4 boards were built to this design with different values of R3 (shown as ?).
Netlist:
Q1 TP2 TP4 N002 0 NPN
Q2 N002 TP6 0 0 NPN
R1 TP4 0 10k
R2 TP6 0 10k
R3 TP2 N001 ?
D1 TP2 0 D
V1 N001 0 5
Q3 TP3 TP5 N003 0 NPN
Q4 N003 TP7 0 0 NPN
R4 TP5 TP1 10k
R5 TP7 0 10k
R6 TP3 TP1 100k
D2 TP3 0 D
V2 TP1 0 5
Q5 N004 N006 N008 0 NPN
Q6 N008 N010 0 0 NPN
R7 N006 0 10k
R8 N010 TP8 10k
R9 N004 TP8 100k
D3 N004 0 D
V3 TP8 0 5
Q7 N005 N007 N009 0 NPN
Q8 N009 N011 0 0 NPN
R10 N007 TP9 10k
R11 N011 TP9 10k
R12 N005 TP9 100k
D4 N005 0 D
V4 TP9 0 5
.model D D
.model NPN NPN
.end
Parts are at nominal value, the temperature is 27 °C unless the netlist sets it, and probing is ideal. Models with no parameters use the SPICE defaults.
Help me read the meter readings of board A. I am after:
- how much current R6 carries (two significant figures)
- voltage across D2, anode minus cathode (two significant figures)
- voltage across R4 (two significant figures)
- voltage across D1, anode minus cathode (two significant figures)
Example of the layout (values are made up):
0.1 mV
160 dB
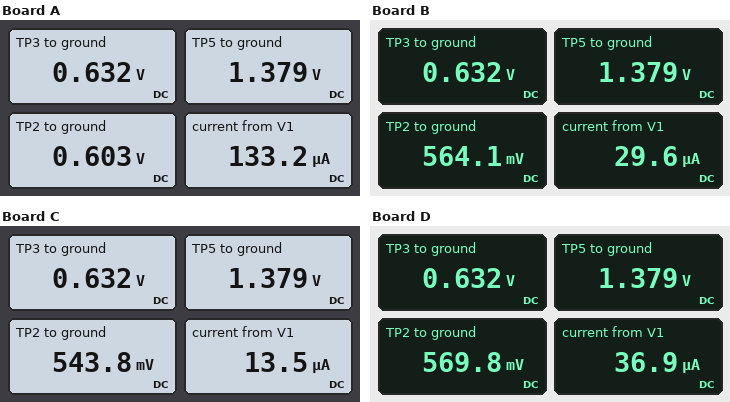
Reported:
44 µA
630 mV
3.6 V
600 mV
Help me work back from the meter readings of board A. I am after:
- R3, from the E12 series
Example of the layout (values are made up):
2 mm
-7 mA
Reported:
33 kΩ
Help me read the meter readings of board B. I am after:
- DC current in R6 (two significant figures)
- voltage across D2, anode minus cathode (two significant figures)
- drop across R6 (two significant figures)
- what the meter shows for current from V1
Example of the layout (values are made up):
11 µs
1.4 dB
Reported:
44 µA
630 mV
4.4 V
29.6 µA
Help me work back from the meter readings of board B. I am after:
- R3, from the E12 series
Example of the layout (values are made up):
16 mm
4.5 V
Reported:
150 kΩ
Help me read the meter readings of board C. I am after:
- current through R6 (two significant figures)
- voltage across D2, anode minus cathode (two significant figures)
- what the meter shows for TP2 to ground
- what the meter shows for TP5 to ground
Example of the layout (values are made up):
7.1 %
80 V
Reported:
44 µA
630 mV
543.8 mV
1.379 V
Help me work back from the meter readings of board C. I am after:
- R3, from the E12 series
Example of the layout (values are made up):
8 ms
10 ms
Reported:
330 kΩ
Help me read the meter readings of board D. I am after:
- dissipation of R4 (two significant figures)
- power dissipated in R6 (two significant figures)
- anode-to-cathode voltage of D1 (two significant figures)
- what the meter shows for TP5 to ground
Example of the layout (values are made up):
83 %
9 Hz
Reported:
1.3 mW
190 µW
570 mV
1.379 V
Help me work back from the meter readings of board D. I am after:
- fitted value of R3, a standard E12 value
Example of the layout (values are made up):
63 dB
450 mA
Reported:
120 kΩ
